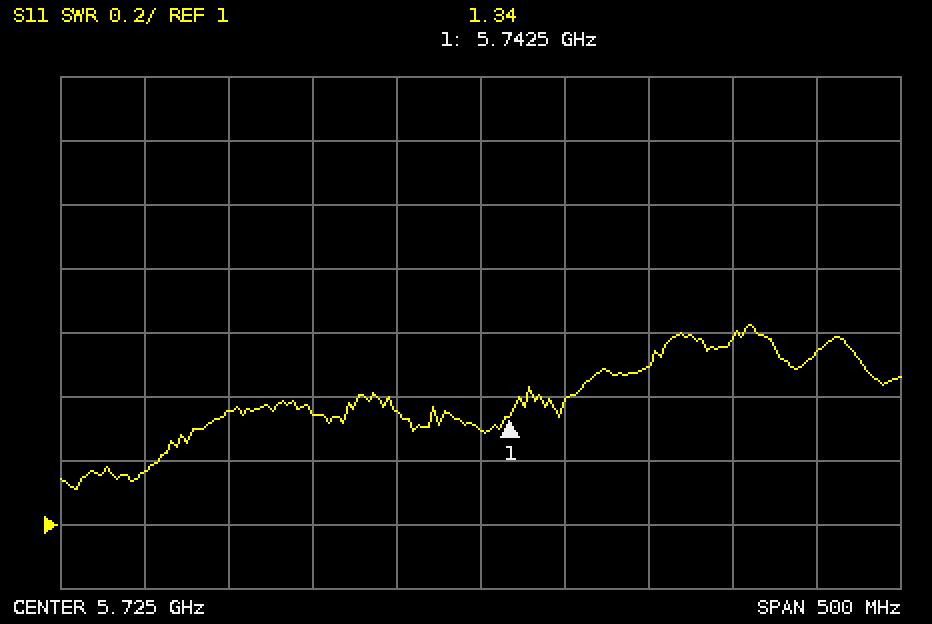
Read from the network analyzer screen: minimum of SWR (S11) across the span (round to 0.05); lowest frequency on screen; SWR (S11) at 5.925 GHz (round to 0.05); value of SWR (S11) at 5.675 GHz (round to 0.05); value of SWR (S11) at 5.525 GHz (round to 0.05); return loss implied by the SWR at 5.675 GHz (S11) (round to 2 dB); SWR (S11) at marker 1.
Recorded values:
1.10
5.475 GHz
1.55
1.35
1.15
16 dB
1.34
